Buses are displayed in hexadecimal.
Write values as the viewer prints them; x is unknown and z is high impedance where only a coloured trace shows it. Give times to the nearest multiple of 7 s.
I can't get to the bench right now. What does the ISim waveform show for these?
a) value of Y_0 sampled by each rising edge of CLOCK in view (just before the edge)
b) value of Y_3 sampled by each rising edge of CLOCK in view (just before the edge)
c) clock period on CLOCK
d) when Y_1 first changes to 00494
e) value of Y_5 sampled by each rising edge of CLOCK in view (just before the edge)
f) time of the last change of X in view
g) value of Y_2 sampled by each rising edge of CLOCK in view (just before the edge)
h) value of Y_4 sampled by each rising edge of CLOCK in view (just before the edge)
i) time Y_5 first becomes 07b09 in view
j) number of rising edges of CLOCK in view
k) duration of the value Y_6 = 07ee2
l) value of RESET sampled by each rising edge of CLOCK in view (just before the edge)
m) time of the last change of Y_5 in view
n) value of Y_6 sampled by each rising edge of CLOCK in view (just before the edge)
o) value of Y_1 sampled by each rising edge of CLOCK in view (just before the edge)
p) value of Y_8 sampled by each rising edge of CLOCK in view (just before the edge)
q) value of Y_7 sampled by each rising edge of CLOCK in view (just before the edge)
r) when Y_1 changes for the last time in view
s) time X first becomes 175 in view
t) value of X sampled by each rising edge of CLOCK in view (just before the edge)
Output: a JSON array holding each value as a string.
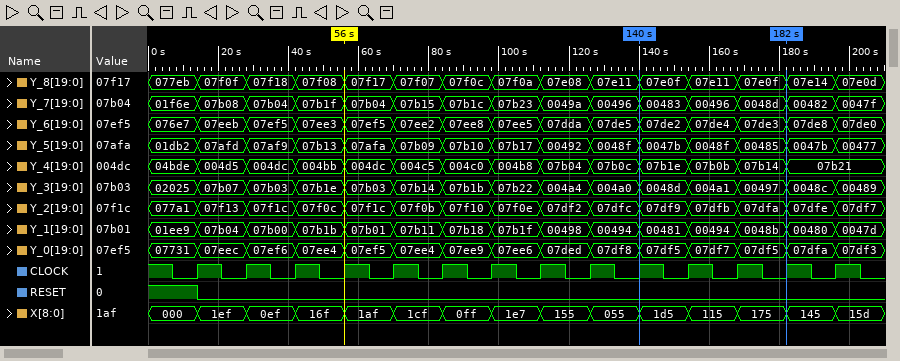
["07731, 07eec, 07ef6, 07ee4, 07ef5, 07ee4, 07ee9, 07ee6, 07ded, 07df8, 07df5, 07df7, 07df5, 07dfa", "02025, 07b07, 07b03, 07b1e, 07b03, 07b14, 07b1b, 07b22, 004a4, 004a0, 0048d, 004a1, 00497, 0048c", "14 s", "126 s", "01db2, 07afd, 07af9, 07b13, 07afa, 07b09, 07b10, 07b17, 00492, 0048f, 0047b, 0048f, 00485, 0047b", "196 s", "077a1, 07f13, 07f1c, 07f0c, 07f1c, 07f0b, 07f10, 07f0e, 07df2, 07dfc, 07df9, 07dfb, 07dfa, 07dfe", "04bde, 004d5, 004dc, 004bb, 004dc, 004c5, 004c0, 004b8, 07b04, 07b0c, 07b1e, 07b0b, 07b14, 07b21", "70 s", "14", "14 s", "1 0 0 0 0 0 0 0 0 0 0 0 0 0", "196 s", "076e7, 07eeb, 07ef5, 07ee3, 07ef5, 07ee2, 07ee8, 07ee5, 07dda, 07de5, 07de2, 07de4, 07de3, 07de8", "01ee9, 07b04, 07b00, 07b1b, 07b01, 07b11, 07b18, 07b1f, 00498, 00494, 00481, 00494, 0048b, 00480", "077eb, 07f0f, 07f18, 07f08, 07f17, 07f07, 07f0c, 07f0a, 07e08, 07e11, 07e0f, 07e11, 07e0f, 07e14", "01f6e, 07b08, 07b04, 07b1f, 07b04, 07b15, 07b1c, 07b23, 0049a, 00496, 00483, 00496, 0048d, 00482", "196 s", "168 s", "000, 1ef, 0ef, 16f, 1af, 1cf, 0ff, 1e7, 155, 055, 1d5, 115, 175, 145"]
